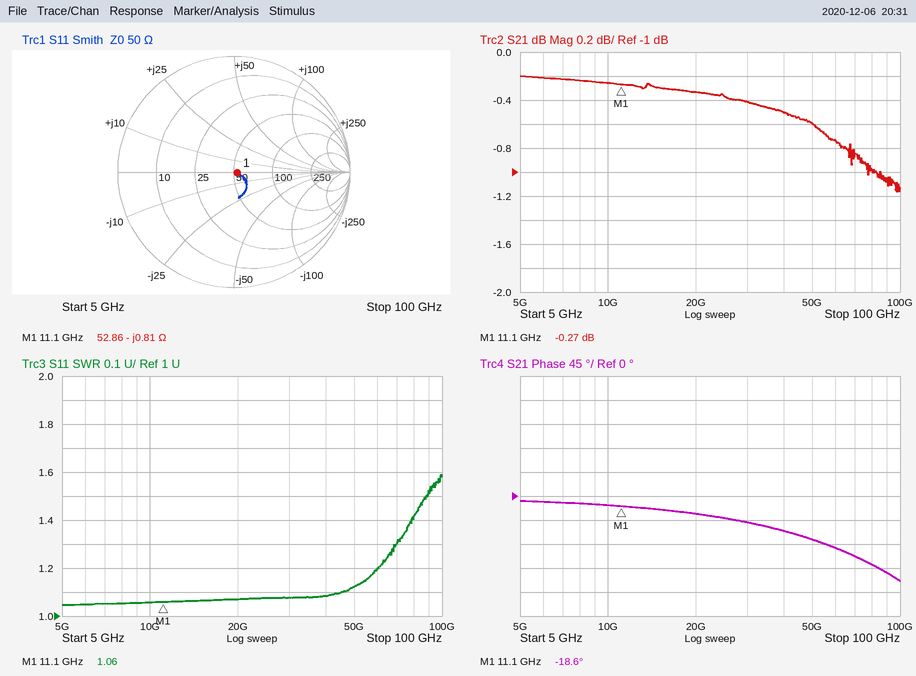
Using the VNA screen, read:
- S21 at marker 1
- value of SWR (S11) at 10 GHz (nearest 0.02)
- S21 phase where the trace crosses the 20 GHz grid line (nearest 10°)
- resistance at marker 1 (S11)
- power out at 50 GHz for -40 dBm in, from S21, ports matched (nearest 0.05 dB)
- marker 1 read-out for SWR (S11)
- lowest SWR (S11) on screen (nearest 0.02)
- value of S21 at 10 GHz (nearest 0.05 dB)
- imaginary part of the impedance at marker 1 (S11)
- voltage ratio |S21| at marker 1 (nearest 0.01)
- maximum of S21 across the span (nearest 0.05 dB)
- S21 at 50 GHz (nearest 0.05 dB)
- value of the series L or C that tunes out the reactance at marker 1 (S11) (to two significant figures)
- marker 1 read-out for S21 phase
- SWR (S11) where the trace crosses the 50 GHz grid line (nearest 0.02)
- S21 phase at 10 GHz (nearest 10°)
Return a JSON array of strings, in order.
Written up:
["-0.27 dB", "1.06", "-30°", "52.86 Ω", "-40.60 dBm", "1.06", "1.04", "-0.25 dB", "-0.81 Ω", "0.97", "-0.20 dB", "-0.60 dB", "12 pH", "-18.6°", "1.12", "-20°"]
